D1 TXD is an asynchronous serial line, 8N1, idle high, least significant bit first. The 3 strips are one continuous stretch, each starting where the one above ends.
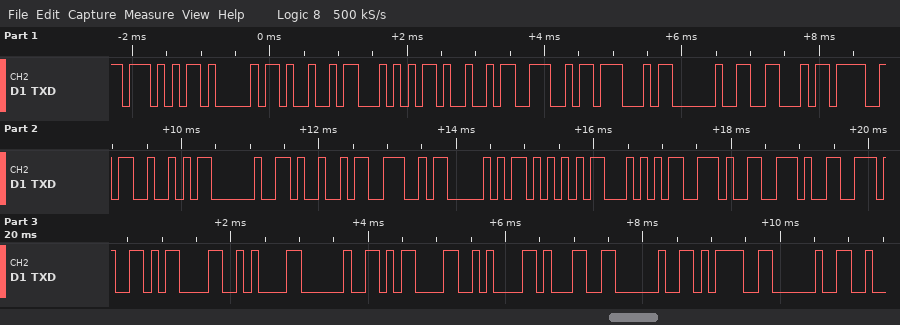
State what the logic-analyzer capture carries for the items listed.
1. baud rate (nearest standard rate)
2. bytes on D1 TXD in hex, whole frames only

9600 baud
57 41 49 54 49 4E 47 20 46 4F 52 20 49 4E 50 55 54 2E 2E 2E 0D 0A 20 0D 0A 31 20 3D 20
